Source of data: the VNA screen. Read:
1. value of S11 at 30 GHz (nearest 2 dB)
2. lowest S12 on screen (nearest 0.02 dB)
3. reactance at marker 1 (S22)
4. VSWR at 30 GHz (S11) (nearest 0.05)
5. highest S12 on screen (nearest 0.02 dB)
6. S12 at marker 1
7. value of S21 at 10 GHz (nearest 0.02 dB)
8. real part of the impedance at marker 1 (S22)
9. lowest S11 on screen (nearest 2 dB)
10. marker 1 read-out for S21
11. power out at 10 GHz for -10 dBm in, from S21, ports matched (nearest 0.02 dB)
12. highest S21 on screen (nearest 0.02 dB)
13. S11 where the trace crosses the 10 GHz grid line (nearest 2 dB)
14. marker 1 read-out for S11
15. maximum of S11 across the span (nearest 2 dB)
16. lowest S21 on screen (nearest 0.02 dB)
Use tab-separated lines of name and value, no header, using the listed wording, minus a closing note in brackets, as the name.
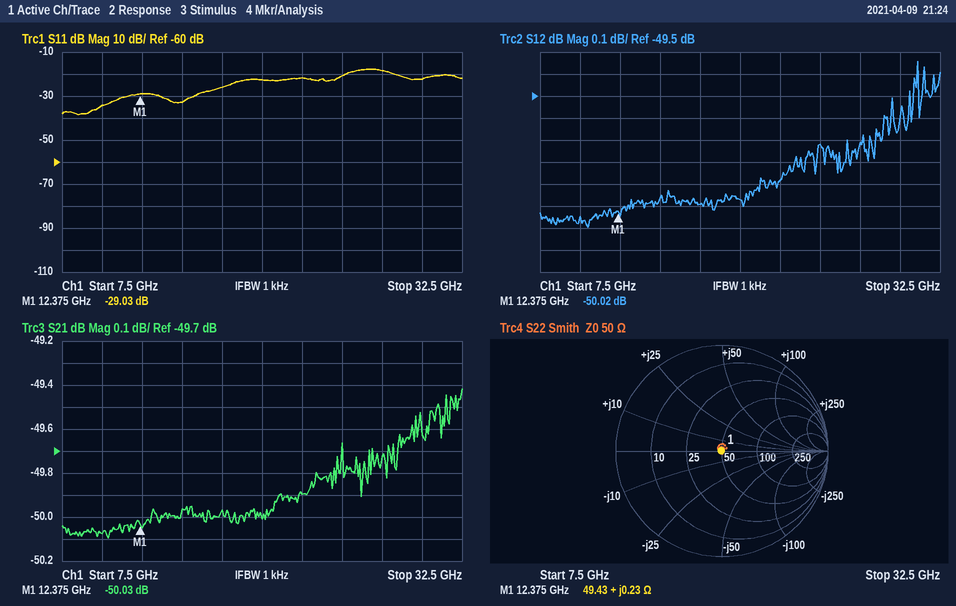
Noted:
value of S11 at 30 GHz	-22 dB
lowest S12 on screen	-50.10 dB
reactance at marker 1	+0.23 Ω
VSWR at 30 GHz (S11)	1.15
highest S12 on screen	-49.34 dB
S12 at marker 1	-50.02 dB
value of S21 at 10 GHz	-50.08 dB
real part of the impedance at marker 1	49.43 Ω
lowest S11 on screen	-38 dB
marker 1 read-out for S21	-50.03 dB
power out at 10 GHz for -10 dBm in, from S21, ports matched	-60.08 dBm
highest S21 on screen	-49.42 dB
S11 where the trace crosses the 10 GHz grid line	-34 dB
marker 1 read-out for S11	-29.03 dB
maximum of S11 across the span	-18 dB
lowest S21 on screen	-50.10 dB
